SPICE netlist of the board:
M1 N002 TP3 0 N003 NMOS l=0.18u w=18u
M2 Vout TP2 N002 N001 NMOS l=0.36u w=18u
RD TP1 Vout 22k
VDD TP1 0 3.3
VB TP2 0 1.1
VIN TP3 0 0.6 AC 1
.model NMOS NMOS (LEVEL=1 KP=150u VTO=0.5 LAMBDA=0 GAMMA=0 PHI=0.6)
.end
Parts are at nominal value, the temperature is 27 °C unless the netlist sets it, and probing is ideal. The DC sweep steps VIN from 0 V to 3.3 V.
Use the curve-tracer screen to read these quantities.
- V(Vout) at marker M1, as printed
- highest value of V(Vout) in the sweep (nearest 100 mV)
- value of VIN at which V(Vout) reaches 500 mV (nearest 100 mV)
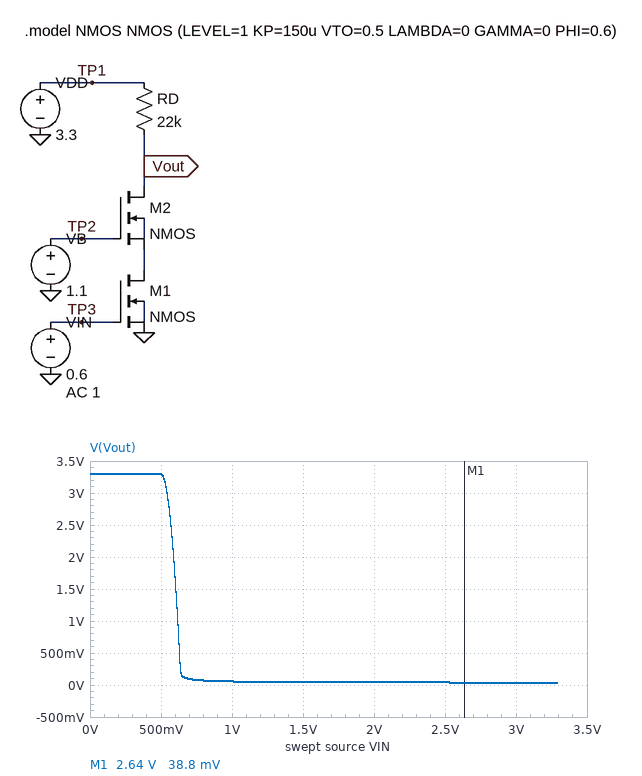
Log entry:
38.8 mV
3.3 V
600 mV
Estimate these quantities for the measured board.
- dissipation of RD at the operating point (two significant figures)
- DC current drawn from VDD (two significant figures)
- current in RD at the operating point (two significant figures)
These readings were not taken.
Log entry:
120 µW
75 µA
75 µA
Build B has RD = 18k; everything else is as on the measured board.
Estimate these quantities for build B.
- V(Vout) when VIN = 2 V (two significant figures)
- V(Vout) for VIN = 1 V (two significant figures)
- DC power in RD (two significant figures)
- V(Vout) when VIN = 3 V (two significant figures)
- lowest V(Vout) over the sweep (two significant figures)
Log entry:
50 mV
68 mV
100 µW
47 mV
46 mV
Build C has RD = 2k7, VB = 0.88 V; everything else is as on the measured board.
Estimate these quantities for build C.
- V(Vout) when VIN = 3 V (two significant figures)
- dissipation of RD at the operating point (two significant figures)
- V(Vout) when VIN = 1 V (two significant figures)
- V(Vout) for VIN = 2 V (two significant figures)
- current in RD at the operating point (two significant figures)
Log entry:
1.9 V
15 µW
2.2 V
2.0 V
75 µA
